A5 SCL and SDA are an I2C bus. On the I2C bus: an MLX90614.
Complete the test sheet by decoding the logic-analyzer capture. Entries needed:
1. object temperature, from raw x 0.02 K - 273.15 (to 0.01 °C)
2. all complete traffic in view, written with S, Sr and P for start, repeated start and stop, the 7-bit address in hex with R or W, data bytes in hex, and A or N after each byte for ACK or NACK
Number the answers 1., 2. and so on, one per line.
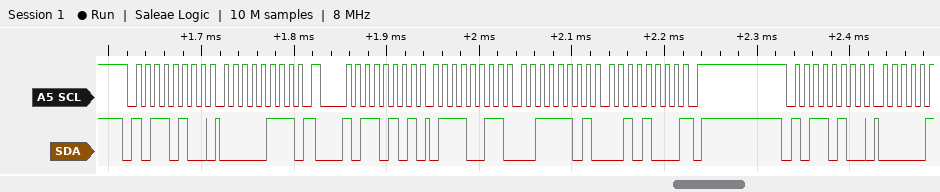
1. 41.47 °C
2. S 5AW A 07 A Sr 5AR A 73 A 3D A 28 N P S 5AW A
